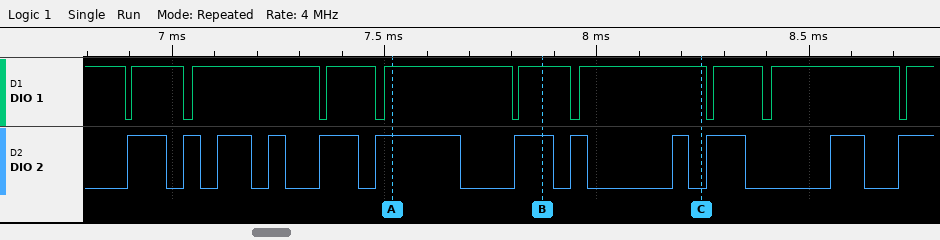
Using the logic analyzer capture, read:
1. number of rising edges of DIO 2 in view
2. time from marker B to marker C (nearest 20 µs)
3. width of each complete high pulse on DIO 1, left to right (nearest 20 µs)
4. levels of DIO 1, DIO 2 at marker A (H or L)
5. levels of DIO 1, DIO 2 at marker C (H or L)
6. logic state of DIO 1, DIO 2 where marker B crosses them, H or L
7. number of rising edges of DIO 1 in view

12
380 µs
120 µs, 300 µs, 120 µs, 300 µs, 120 µs, 300 µs, 120 µs, 300 µs
DIO 1=H, DIO 2=H
DIO 1=H, DIO 2=L
DIO 1=H, DIO 2=H
9
